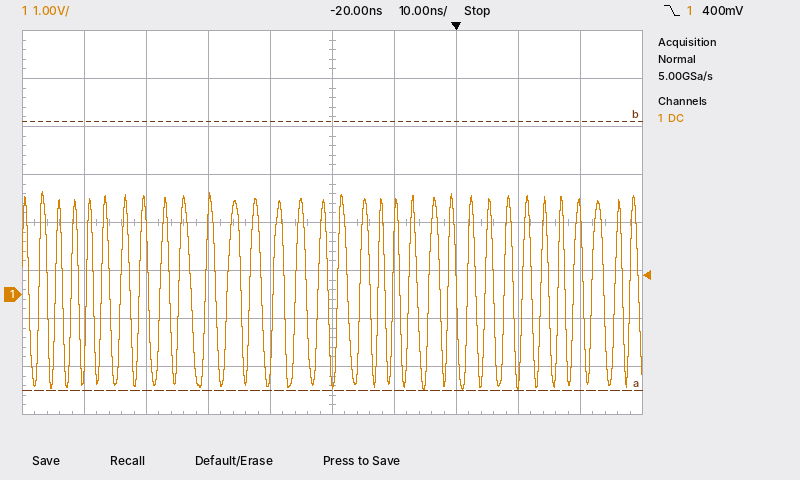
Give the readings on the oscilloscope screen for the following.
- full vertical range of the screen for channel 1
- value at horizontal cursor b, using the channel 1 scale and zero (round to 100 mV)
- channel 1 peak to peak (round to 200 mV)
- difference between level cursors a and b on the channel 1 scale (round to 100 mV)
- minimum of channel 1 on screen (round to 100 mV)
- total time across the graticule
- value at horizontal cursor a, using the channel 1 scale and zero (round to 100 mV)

8 V
3.6 V
4.2 V
5.6 V
-2.0 V
100 ns
-2.0 V
